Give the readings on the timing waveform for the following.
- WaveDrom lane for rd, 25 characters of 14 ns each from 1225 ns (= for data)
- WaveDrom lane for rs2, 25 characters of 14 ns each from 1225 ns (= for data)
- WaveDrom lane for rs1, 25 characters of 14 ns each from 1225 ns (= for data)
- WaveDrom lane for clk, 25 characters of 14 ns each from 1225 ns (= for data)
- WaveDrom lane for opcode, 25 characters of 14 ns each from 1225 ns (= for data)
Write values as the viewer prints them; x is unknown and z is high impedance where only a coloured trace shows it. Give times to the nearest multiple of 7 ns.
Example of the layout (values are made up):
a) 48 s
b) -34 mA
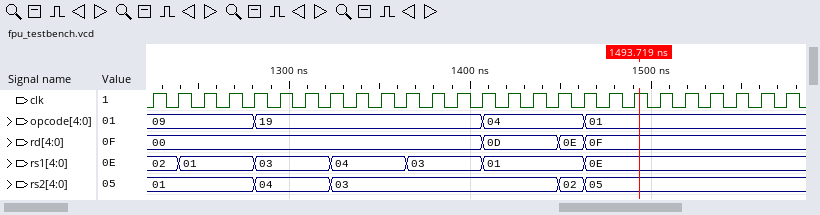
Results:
a) {name: 'rd', wave: '=............=..==.......', data: '00 0D 0E 0F'}
b) {name: 'rs2', wave: '=...=..=........==.......', data: '01 04 03 02 05'}
c) {name: 'rs1', wave: '==..=..=..=..=...=.......', data: '02 01 03 04 03 01 0E'}
d) {name: 'clk', wave: 'p........................'}
e) {name: 'opcode', wave: '=...=........=...=.......', data: '09 19 04 01'}
